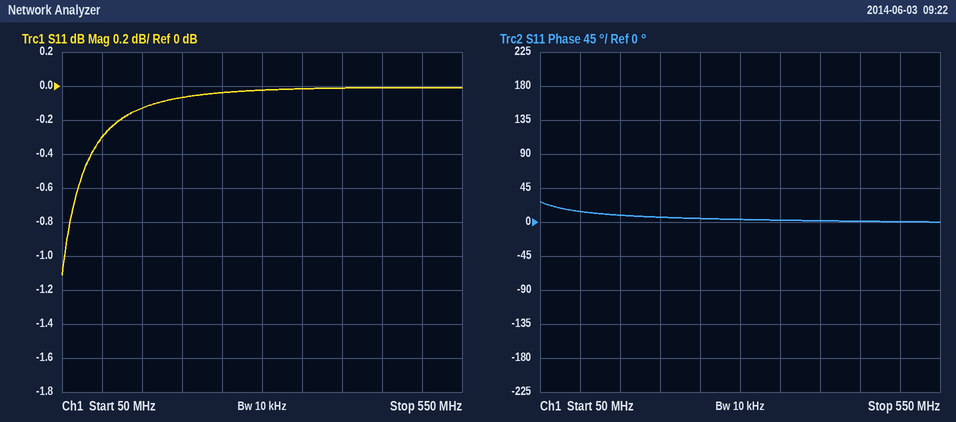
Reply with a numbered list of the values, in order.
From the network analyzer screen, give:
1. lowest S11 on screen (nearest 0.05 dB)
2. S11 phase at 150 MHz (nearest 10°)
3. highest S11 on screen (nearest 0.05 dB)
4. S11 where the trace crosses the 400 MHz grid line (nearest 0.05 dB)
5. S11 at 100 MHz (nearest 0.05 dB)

1. -1.10 dB
2. 10°
3. 0.00 dB
4. 0.00 dB
5. -0.30 dB
